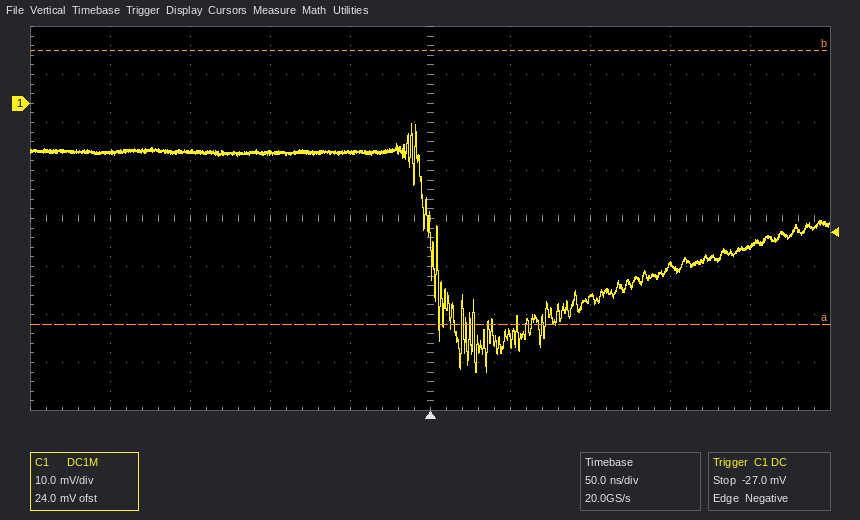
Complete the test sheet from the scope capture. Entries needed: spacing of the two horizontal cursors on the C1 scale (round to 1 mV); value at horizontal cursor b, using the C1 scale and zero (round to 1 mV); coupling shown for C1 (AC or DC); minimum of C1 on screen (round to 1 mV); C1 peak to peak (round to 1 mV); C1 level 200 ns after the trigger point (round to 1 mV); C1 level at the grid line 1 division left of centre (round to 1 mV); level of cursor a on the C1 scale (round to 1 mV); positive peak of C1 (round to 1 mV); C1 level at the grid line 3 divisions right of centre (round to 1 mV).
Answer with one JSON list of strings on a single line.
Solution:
["57 mV", "11 mV", "DC", "-56 mV", "52 mV", "-30 mV", "-10 mV", "-46 mV", "-4 mV", "-34 mV"]
